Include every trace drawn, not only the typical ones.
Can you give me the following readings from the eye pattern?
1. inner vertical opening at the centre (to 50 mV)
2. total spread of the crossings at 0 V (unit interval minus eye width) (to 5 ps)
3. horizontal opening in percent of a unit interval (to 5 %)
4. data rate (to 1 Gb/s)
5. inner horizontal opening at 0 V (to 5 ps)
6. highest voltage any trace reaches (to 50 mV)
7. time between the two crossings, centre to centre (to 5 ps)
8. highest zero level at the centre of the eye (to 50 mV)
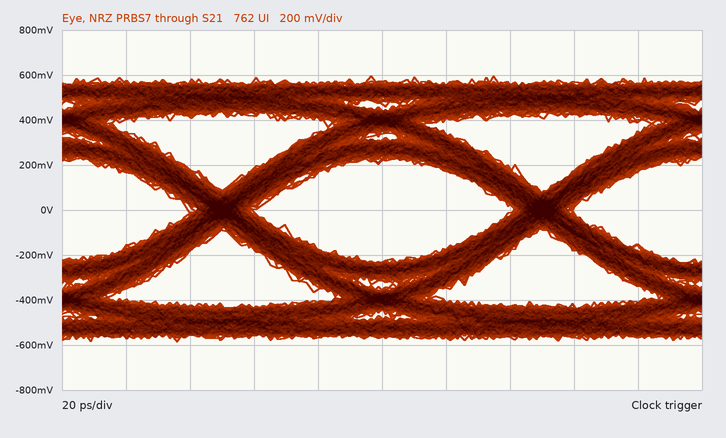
450 mV
20 ps
80 %
10 Gb/s
80 ps
600 mV
100 ps
-250 mV
